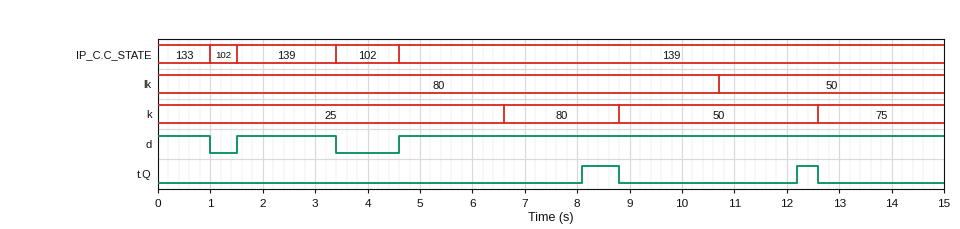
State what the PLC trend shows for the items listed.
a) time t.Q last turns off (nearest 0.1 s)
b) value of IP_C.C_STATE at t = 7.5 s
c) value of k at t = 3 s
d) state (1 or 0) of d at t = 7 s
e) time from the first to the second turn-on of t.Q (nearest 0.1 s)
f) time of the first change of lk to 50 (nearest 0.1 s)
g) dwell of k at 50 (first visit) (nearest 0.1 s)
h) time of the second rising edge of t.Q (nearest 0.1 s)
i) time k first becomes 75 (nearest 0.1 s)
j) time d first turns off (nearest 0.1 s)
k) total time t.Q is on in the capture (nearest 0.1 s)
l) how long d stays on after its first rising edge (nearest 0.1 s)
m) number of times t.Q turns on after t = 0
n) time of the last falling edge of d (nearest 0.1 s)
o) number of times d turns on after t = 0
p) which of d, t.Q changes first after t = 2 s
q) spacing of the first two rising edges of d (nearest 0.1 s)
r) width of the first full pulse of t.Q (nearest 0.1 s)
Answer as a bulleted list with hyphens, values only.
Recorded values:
- 12.6 s
- 139
- 25
- 1
- 4.1 s
- 10.7 s
- 3.8 s
- 12.2 s
- 12.6 s
- 1.0 s
- 1.1 s
- 1.9 s
- 2
- 3.4 s
- 2
- d
- 3.1 s
- 0.7 s
